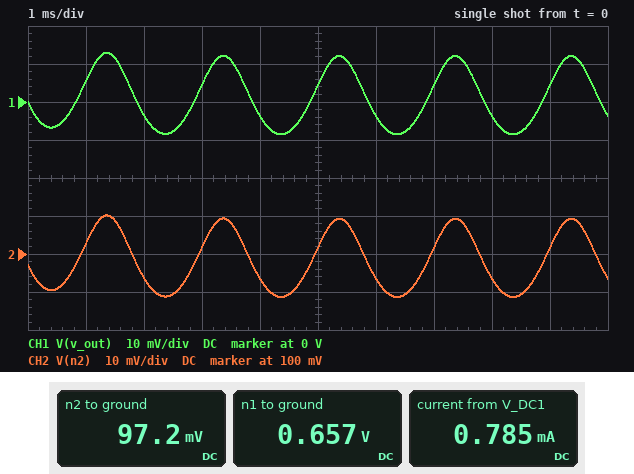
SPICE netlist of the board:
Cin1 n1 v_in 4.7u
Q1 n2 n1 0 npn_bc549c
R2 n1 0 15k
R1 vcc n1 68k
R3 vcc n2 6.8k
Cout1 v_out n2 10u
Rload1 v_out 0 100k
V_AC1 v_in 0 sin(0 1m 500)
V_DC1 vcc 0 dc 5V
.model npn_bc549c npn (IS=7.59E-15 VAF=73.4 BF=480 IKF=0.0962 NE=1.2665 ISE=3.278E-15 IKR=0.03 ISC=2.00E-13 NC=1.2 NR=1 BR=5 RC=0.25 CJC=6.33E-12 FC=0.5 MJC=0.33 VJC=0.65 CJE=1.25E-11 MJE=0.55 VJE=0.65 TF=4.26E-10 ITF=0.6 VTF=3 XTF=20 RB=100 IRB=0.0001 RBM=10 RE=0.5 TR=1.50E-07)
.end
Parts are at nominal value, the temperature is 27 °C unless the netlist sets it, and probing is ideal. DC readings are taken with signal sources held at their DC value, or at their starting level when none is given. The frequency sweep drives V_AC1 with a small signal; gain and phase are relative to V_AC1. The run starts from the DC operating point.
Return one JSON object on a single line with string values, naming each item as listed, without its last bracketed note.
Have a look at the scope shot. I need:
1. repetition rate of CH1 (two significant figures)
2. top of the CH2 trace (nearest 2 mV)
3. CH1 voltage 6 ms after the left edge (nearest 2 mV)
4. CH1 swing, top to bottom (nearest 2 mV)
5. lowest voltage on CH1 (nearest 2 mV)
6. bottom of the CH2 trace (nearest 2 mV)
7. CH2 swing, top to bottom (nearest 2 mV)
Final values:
{"repetition rate of CH1": "500 Hz", "top of the CH2 trace": "110 mV", "CH1 voltage 6 ms after the left edge": "-4 mV", "CH1 swing, top to bottom": "22 mV", "lowest voltage on CH1": "-8 mV", "bottom of the CH2 trace": "88 mV", "CH2 swing, top to bottom": "22 mV"}
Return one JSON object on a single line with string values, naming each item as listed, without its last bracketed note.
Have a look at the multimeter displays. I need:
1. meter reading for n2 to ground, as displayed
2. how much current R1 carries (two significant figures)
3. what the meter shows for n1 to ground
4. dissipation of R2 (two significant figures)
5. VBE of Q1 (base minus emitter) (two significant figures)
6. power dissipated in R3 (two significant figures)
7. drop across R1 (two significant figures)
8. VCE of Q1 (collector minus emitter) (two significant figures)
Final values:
{"meter reading for n2 to ground, as displayed": "97.2 mV", "how much current R1 carries": "64 µA", "what the meter shows for n1 to ground": "0.657 V", "dissipation of R2": "29 µW", "VBE of Q1 (base minus emitter)": "660 mV", "power dissipated in R3": "3.5 mW", "drop across R1": "4.3 V", "VCE of Q1 (collector minus emitter)": "97 mV"}
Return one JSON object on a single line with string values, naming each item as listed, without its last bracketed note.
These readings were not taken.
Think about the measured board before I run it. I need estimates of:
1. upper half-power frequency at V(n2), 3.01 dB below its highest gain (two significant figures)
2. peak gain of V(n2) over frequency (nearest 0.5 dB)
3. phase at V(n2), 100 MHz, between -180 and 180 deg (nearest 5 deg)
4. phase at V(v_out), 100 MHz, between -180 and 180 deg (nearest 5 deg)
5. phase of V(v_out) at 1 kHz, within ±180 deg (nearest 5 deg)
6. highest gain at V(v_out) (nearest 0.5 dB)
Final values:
{"upper half-power frequency at V(n2), 3.01 dB below its highest gain": "1.1 MHz", "peak gain of V(n2) over frequency": "20.0 dB", "phase at V(n2), 100 MHz, between -180 and 180 deg": "-10 deg", "phase at V(v_out), 100 MHz, between -180 and 180 deg": "-10 deg", "phase of V(v_out) at 1 kHz, within ±180 deg": "-170 deg", "highest gain at V(v_out)": "20.0 dB"}
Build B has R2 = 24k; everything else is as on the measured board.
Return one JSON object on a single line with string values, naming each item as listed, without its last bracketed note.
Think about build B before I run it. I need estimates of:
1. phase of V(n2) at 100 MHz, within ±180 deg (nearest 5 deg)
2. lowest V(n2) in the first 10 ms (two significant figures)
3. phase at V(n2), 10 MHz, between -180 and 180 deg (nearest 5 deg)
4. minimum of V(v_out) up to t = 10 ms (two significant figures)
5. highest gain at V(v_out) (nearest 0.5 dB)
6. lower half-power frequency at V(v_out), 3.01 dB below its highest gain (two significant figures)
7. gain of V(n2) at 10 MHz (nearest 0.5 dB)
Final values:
{"phase of V(n2) at 100 MHz, within ±180 deg": "-20 deg", "lowest V(n2) in the first 10 ms": "74 mV", "phase at V(n2), 10 MHz, between -180 and 180 deg": "65 deg", "minimum of V(v_out) up to t = 10 ms": "-4.8 mV", "highest gain at V(v_out)": "14.5 dB", "lower half-power frequency at V(v_out), 3.01 dB below its highest gain": "220 Hz", "gain of V(n2) at 10 MHz": "-3.5 dB"}
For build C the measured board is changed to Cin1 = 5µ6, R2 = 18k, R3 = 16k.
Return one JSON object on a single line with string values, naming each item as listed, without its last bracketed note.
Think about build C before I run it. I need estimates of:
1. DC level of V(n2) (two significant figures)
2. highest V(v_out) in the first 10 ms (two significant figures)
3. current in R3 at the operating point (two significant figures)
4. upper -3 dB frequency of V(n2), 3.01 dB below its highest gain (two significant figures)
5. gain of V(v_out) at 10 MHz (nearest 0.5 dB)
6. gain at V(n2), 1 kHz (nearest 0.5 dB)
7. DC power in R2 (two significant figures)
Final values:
{"DC level of V(n2)": "64 mV", "highest V(v_out) in the first 10 ms": "4.6 mV", "current in R3 at the operating point": "310 µA", "upper -3 dB frequency of V(n2), 3.01 dB below its highest gain": "1.3 MHz", "gain of V(v_out) at 10 MHz": "-3.5 dB", "gain at V(n2), 1 kHz": "11.5 dB", "DC power in R2": "23 µW"}
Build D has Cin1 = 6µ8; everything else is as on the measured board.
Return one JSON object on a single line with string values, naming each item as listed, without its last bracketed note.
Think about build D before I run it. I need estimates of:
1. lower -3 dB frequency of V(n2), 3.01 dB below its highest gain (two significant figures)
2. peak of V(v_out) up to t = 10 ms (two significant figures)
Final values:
{"lower -3 dB frequency of V(n2), 3.01 dB below its highest gain": "140 Hz", "peak of V(v_out) up to t = 10 ms": "14 mV"}
